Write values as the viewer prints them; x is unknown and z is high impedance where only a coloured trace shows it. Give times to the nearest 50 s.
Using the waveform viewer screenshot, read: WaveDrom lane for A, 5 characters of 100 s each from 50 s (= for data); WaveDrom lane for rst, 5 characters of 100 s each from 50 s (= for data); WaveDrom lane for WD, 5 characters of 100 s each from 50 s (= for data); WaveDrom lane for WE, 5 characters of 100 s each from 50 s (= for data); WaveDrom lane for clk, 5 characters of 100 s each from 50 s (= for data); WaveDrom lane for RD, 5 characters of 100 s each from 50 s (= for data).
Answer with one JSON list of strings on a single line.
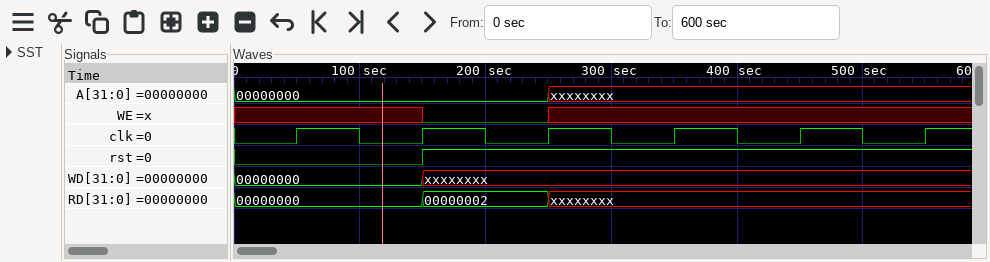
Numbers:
["{name: 'A', wave: '=.x..', data: '00000000'}", "{name: 'rst', wave: '01...'}", "{name: 'WD', wave: '=x...', data: '00000000'}", "{name: 'WE', wave: 'x0x..'}", "{name: 'clk', wave: 'p....'}", "{name: 'RD', wave: '==x..', data: '00000000 00000002'}"]
